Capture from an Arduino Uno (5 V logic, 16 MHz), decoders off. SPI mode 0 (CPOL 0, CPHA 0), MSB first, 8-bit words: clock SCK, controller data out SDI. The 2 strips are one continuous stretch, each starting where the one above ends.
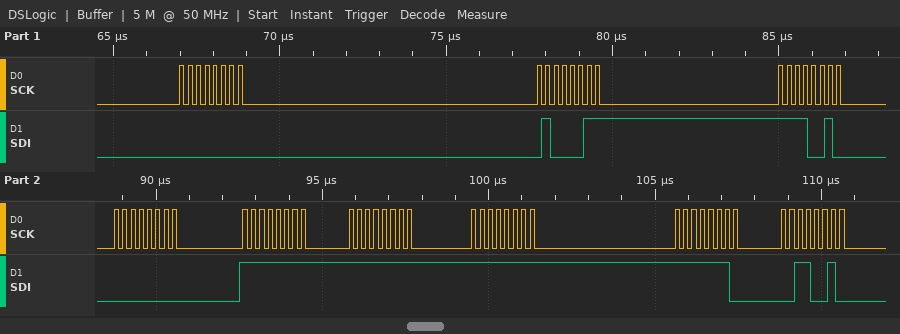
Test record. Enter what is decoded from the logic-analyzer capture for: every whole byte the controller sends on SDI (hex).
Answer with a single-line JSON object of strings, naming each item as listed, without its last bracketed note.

{"every whole byte the controller sends on SDI": "0x00 0x43 0xF2 0x00 0xFF 0xFF 0xFF 0xFE 0x32"}
